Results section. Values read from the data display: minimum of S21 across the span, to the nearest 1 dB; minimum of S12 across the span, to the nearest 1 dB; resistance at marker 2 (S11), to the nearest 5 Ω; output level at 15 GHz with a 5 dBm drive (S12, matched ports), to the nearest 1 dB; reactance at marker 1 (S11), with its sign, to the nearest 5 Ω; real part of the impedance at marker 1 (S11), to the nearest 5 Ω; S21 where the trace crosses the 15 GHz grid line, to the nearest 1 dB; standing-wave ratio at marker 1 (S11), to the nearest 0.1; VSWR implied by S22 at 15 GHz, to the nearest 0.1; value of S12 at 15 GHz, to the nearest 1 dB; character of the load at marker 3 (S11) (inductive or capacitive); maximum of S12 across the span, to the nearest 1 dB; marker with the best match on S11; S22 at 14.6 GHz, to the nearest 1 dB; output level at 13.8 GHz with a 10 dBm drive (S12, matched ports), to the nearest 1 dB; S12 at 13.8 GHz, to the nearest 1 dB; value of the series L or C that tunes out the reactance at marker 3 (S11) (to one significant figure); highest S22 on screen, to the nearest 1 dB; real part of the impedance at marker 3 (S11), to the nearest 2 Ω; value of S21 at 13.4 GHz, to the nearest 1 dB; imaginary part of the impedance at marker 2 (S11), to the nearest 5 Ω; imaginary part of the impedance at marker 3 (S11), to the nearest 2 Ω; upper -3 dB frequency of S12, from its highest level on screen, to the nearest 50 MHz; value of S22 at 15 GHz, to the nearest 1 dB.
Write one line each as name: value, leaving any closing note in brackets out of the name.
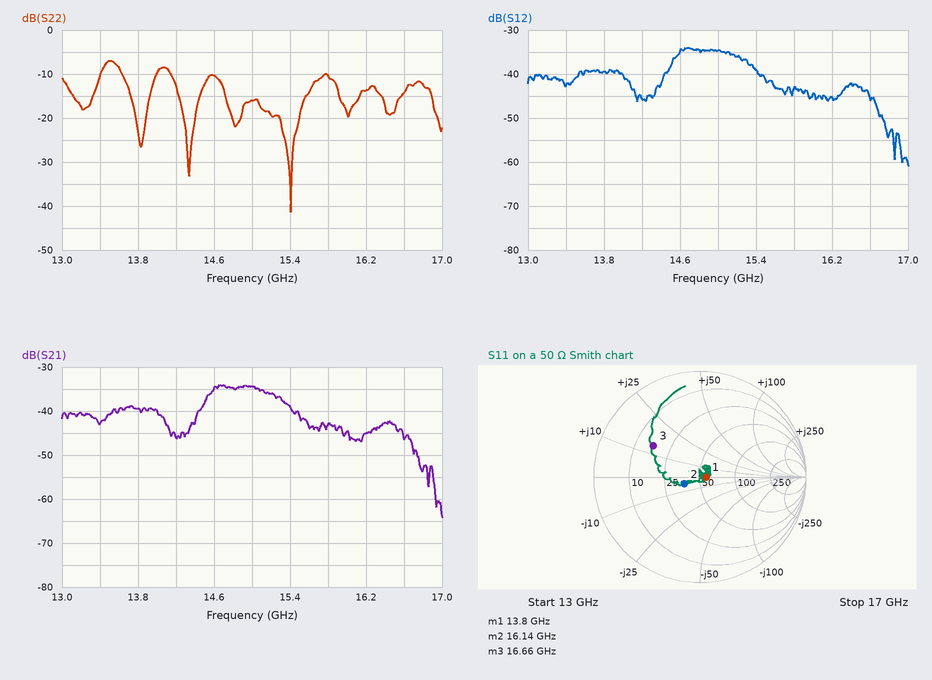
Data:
minimum of S21 across the span, to the nearest 1 dB: -64 dB
minimum of S12 across the span, to the nearest 1 dB: -61 dB
resistance at marker 2 (S11), to the nearest 5 Ω: 35 Ω
output level at 15 GHz with a 5 dBm drive (S12, matched ports), to the nearest 1 dB: -30 dBm
reactance at marker 1 (S11), with its sign, to the nearest 5 Ω: 0 Ω
real part of the impedance at marker 1 (S11), to the nearest 5 Ω: 55 Ω
S21 where the trace crosses the 15 GHz grid line, to the nearest 1 dB: -34 dB
standing-wave ratio at marker 1 (S11), to the nearest 0.1: 1.1
VSWR implied by S22 at 15 GHz, to the nearest 0.1: 1.4
value of S12 at 15 GHz, to the nearest 1 dB: -35 dB
character of the load at marker 3 (S11): inductive
maximum of S12 across the span, to the nearest 1 dB: -34 dB
marker with the best match on S11: marker 1
S22 at 14.6 GHz, to the nearest 1 dB: -10 dB
output level at 13.8 GHz with a 10 dBm drive (S12, matched ports), to the nearest 1 dB: -29 dBm
S12 at 13.8 GHz, to the nearest 1 dB: -39 dB
value of the series L or C that tunes out the reactance at marker 3 (S11): 700 fF
highest S22 on screen, to the nearest 1 dB: -7 dB
real part of the impedance at marker 3 (S11), to the nearest 2 Ω: 16 Ω
value of S21 at 13.4 GHz, to the nearest 1 dB: -43 dB
imaginary part of the impedance at marker 2 (S11), to the nearest 5 Ω: -5 Ω
imaginary part of the impedance at marker 3 (S11), to the nearest 2 Ω: +14 Ω
upper -3 dB frequency of S12, from its highest level on screen, to the nearest 50 MHz: 15.30 GHz
value of S22 at 15 GHz, to the nearest 1 dB: -16 dB
